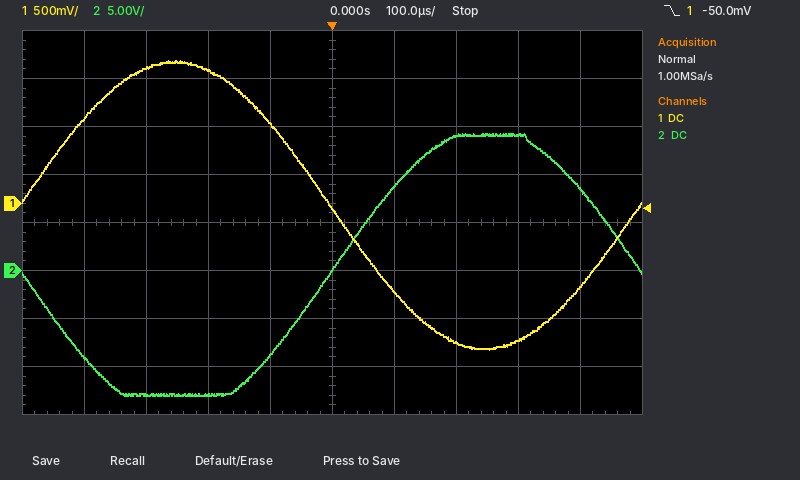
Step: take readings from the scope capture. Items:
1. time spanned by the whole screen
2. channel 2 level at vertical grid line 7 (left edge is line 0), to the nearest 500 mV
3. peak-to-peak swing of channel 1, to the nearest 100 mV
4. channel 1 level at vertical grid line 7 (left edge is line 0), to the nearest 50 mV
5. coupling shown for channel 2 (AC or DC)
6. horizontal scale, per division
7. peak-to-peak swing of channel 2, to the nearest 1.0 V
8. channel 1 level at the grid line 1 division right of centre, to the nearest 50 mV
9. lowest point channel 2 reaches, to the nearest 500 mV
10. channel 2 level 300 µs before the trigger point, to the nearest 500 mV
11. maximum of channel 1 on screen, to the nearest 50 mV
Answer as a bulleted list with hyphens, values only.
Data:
- 1 ms
- 14.0 V
- 3.00 V
- -1.45 V
- DC
- 100 µs
- 27.0 V
- -900 mV
- -13.0 V
- -13.0 V
- 1.50 V
